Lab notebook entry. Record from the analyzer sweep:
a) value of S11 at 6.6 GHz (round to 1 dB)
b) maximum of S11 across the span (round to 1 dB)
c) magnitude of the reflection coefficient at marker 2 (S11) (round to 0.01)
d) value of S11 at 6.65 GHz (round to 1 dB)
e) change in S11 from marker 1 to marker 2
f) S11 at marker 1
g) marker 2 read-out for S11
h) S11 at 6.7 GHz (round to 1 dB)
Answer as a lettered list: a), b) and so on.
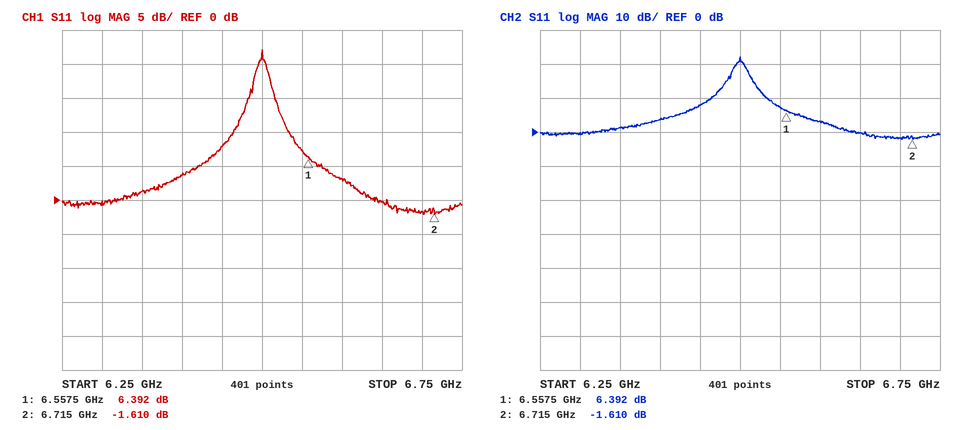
a) 3 dB
b) 22 dB
c) 0.83
d) 0 dB
e) -8.002 dB
f) 6.392 dB
g) -1.610 dB
h) -2 dB
